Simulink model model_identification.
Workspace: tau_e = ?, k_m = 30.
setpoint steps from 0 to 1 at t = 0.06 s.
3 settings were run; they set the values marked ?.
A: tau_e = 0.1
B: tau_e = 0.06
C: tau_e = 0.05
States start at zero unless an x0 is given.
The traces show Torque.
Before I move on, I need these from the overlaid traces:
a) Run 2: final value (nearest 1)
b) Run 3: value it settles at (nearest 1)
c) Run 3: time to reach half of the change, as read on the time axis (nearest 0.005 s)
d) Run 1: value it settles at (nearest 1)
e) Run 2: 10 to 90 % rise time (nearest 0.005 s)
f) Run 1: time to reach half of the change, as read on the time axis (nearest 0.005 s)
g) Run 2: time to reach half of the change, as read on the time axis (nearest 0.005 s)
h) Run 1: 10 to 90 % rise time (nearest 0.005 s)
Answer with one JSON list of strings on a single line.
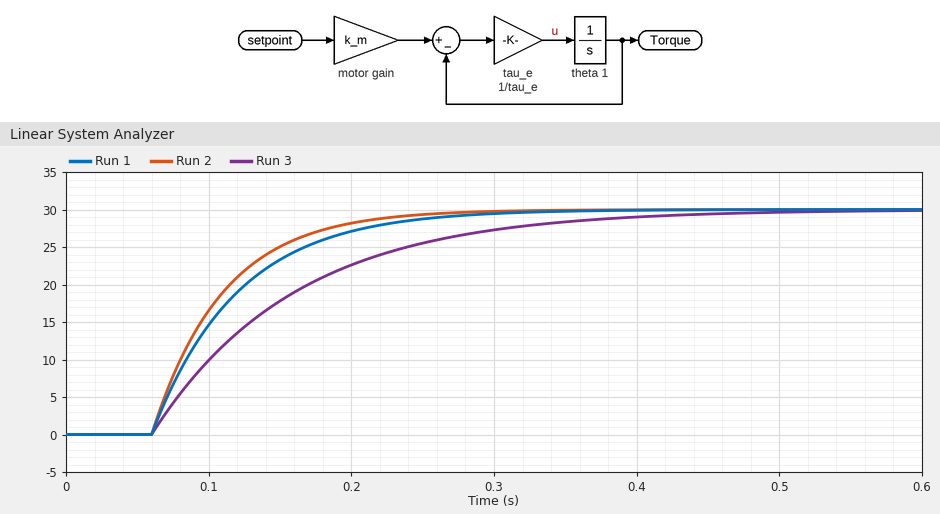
["30", "30", "0.130 s", "30", "0.110 s", "0.100 s", "0.095 s", "0.130 s"]
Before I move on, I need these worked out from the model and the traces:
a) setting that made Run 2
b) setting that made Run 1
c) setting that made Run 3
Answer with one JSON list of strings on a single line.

["C", "B", "A"]
